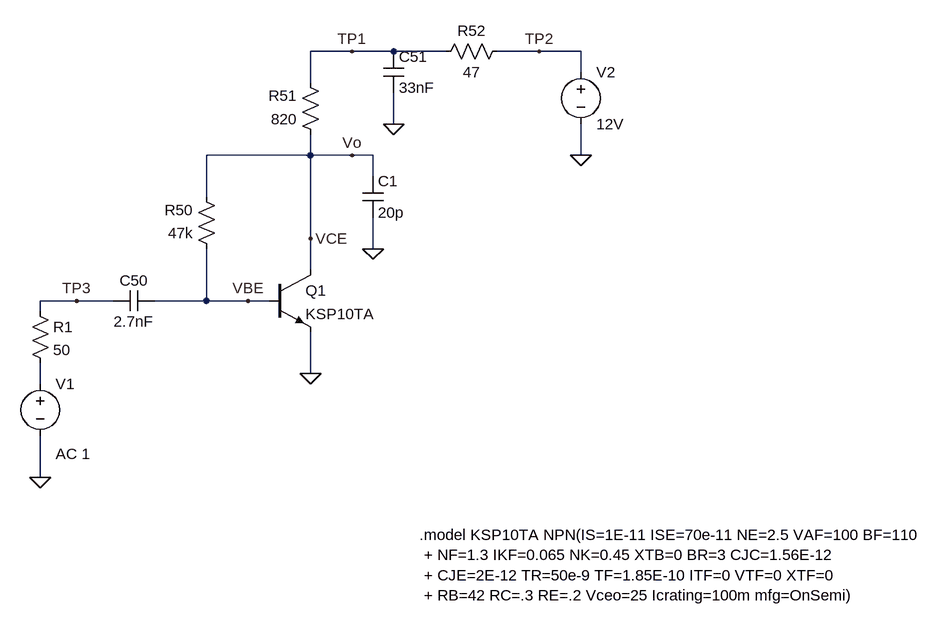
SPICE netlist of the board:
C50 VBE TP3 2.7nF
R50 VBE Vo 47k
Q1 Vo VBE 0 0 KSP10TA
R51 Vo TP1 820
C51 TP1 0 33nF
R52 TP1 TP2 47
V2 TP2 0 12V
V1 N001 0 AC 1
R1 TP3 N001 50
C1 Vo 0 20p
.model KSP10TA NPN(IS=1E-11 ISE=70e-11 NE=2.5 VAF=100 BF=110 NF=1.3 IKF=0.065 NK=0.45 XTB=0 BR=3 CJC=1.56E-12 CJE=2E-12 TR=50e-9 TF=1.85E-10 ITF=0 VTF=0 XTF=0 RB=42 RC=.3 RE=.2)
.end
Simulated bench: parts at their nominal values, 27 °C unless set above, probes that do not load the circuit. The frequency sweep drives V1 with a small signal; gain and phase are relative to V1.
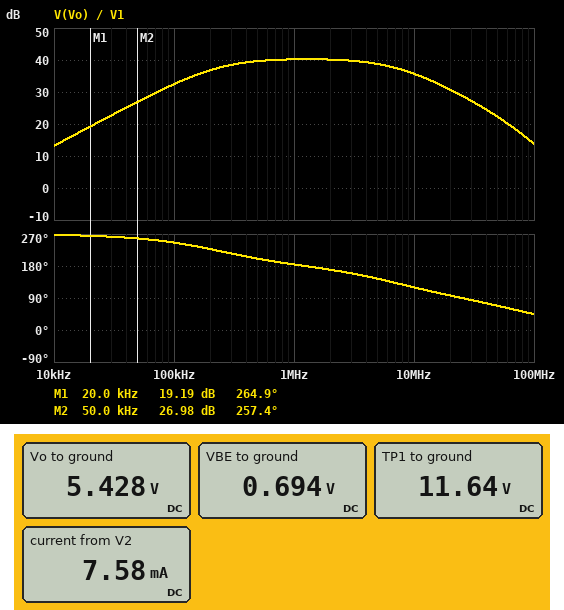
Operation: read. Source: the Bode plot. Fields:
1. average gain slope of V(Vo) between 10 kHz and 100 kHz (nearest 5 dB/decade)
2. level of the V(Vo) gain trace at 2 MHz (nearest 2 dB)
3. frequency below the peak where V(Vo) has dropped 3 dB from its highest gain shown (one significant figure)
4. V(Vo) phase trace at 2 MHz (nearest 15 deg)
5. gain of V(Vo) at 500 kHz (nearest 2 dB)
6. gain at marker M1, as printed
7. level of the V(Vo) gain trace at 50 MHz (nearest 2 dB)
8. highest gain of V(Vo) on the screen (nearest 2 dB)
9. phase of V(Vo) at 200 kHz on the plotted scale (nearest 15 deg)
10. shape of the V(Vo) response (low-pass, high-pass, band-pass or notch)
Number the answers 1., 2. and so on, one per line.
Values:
1. 20 dB/decade
2. 40 dB
3. 200 kHz
4. 165 deg
5. 40 dB
6. 19.19 dB
7. 22 dB
8. 40 dB
9. 225 deg
10. band-pass
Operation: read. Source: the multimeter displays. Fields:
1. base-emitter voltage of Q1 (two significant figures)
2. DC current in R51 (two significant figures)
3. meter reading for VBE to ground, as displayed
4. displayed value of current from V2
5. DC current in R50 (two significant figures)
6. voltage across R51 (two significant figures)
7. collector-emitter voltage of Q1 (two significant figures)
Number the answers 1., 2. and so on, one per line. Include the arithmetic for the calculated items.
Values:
1. 694 mV = 690 mV
2. (11.64 V - 5.428 V) / 820 Ω = 7.6 mA
3. 0.694 V
4. 7.58 mA
5. (5.428 V - 694 mV) / 47 kΩ = 100 µA
6. 11.64 V - 5.428 V = 6.2 V
7. 5.428 V = 5.4 V
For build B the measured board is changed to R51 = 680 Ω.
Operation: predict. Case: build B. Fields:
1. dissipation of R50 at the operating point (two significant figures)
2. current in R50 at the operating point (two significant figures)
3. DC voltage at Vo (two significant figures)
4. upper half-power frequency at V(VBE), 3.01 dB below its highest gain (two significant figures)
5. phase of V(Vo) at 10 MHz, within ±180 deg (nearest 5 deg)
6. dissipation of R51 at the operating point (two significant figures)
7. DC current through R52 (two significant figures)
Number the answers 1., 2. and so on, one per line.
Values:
1. 570 µW
2. 110 µA
3. 5.9 V
4. 120 MHz
5. 125 deg
6. 48 mW
7. 8.4 mA
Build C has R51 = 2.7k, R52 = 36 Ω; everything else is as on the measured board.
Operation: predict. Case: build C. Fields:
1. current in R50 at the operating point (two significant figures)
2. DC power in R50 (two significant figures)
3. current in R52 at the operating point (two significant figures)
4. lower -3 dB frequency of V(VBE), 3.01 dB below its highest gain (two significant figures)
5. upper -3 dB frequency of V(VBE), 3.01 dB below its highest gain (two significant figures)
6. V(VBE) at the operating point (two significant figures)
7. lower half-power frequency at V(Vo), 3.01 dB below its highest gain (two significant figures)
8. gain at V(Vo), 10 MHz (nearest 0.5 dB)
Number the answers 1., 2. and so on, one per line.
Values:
1. 49 µA
2. 110 µW
3. 3.3 mA
4. 270 kHz
5. 210 MHz
6. 660 mV
7. 220 kHz
8. 33.0 dB
